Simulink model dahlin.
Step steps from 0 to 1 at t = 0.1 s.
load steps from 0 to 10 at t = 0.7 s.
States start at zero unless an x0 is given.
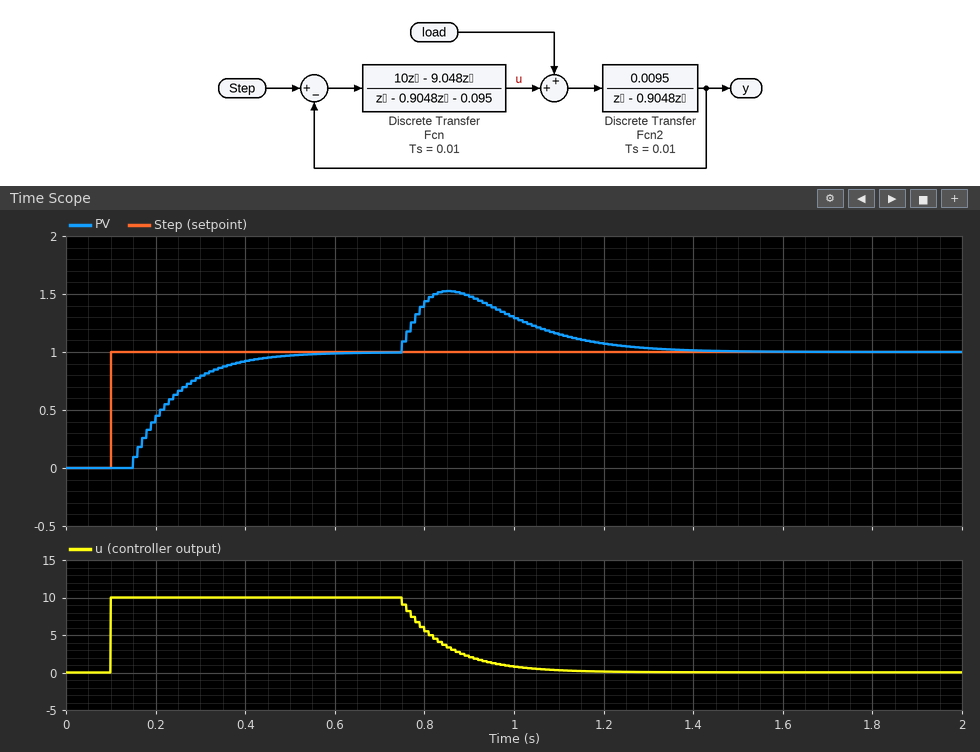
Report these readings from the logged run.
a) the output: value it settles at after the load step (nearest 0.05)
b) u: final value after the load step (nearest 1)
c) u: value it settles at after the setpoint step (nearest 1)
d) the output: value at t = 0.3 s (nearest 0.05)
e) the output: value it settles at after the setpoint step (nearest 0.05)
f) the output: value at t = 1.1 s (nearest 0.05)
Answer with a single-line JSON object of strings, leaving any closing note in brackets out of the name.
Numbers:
{"the output: value it settles at after the load step": "1.00", "u: final value after the load step": "0", "u: value it settles at after the setpoint step": "10", "the output: value at t = 0.3 s": "0.80", "the output: value it settles at after the setpoint step": "1.00", "the output: value at t = 1.1 s": "1.15"}
